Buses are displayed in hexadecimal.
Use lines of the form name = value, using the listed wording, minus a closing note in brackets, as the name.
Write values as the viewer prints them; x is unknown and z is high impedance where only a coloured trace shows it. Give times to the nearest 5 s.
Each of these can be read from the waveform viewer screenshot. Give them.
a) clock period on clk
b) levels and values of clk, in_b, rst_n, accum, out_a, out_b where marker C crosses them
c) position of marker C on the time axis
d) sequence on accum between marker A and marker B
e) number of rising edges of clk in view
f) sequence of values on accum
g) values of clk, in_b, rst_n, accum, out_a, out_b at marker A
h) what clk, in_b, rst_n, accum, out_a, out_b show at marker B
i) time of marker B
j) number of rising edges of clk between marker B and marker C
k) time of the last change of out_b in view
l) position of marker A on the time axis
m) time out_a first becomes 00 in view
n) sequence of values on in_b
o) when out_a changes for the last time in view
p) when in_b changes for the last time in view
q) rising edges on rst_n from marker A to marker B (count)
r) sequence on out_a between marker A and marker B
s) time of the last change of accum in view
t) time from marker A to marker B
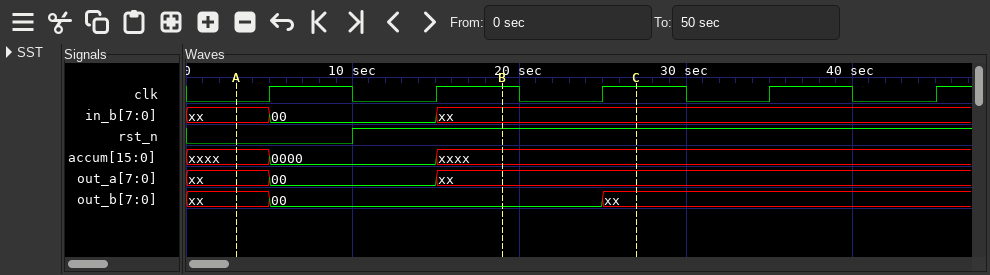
clock period on clk = 10 s
levels and values of clk, in_b, rst_n, accum, out_a, out_b where marker C crosses them = clk=1, in_b=xx, rst_n=1, accum=xxxx, out_a=xx, out_b=xx
position of marker C on the time axis = 25 s
sequence on accum between marker A and marker B = xxxx, 0000, xxxx
number of rising edges of clk in view = 5
sequence of values on accum = xxxx, 0000, xxxx
values of clk, in_b, rst_n, accum, out_a, out_b at marker A = clk=0, in_b=xx, rst_n=0, accum=xxxx, out_a=xx, out_b=xx
what clk, in_b, rst_n, accum, out_a, out_b show at marker B = clk=1, in_b=xx, rst_n=1, accum=xxxx, out_a=xx, out_b=00
time of marker B = 20 s
number of rising edges of clk between marker B and marker C = 1
time of the last change of out_b in view = 25 s
position of marker A on the time axis = 5 s
time out_a first becomes 00 in view = 5 s
sequence of values on in_b = xx, 00, xx
when out_a changes for the last time in view = 15 s
when in_b changes for the last time in view = 15 s
rising edges on rst_n from marker A to marker B = 1
sequence on out_a between marker A and marker B = xx, 00, xx
time of the last change of accum in view = 15 s
time from marker A to marker B = 15 s
